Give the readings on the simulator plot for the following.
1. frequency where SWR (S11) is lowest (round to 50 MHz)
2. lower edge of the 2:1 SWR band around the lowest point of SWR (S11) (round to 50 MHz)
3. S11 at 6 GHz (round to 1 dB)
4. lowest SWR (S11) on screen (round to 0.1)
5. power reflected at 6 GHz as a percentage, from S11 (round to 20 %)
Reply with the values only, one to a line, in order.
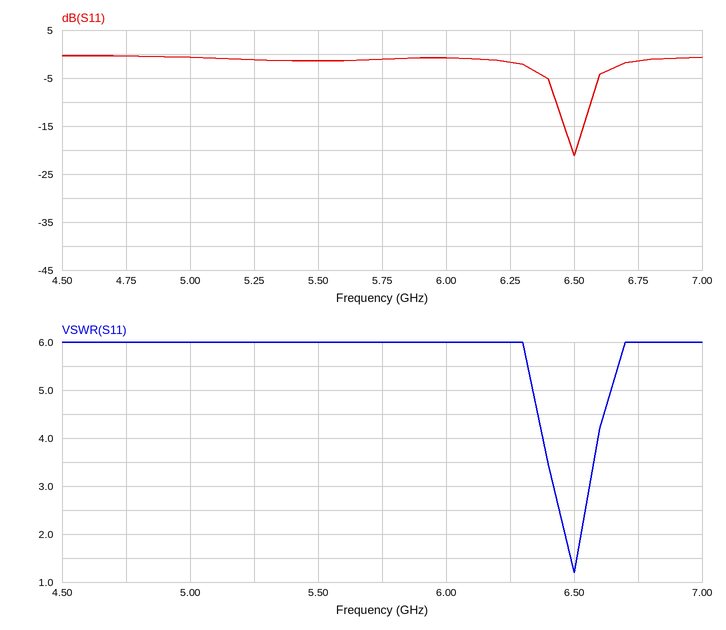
6.50 GHz
6.45 GHz
-1 dB
1.2
80 %
